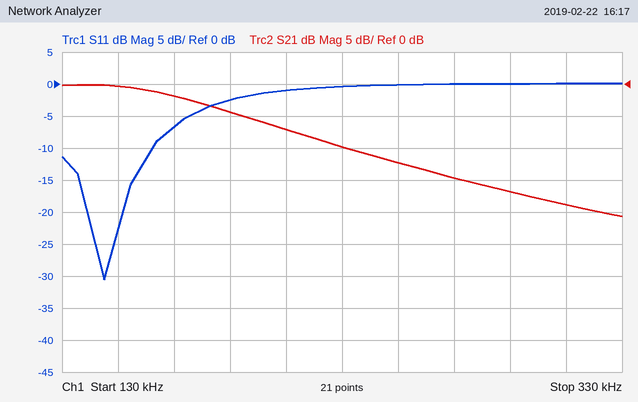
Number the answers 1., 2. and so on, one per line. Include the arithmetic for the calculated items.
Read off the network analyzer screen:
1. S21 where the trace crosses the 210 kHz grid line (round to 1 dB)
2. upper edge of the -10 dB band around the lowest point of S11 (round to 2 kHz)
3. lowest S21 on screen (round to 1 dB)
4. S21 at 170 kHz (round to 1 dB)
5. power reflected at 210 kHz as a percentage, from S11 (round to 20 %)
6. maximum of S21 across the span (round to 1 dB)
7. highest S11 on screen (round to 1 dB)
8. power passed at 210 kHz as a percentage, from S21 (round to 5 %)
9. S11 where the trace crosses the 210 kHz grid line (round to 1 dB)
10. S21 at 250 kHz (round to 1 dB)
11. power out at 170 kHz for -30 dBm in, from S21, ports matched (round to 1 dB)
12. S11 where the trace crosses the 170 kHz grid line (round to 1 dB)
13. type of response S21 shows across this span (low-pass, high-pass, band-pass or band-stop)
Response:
1. -7 dB
2. 162 kHz
3. -21 dB
4. -2 dB
5. 10^(-1/10) ≈ 79.4 %, so 80 % to the nearest 20 %
6. 0 dB
7. 0 dB
8. 10^(-7/10) ≈ 20 %
9. -1 dB
10. -12 dB
11. -30 dBm + (-2 dB) = -32 dBm
12. -7 dB
13. low-pass
